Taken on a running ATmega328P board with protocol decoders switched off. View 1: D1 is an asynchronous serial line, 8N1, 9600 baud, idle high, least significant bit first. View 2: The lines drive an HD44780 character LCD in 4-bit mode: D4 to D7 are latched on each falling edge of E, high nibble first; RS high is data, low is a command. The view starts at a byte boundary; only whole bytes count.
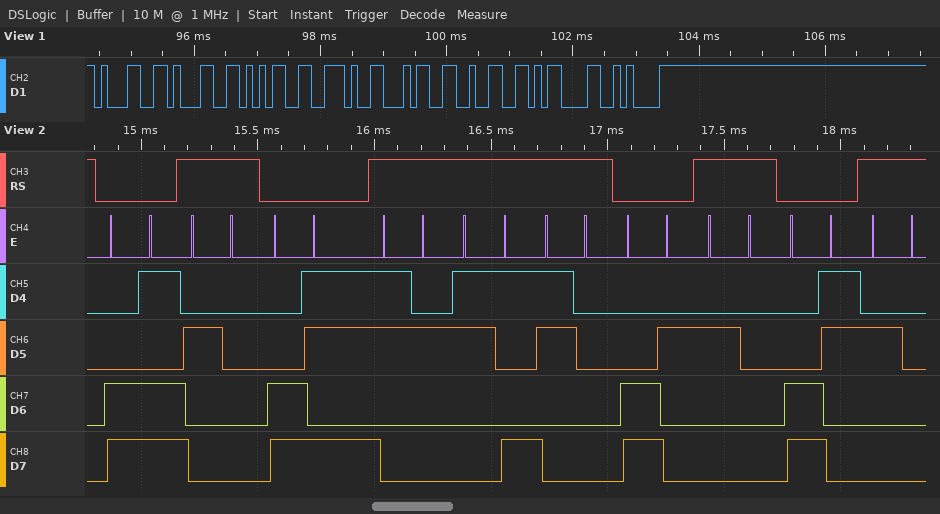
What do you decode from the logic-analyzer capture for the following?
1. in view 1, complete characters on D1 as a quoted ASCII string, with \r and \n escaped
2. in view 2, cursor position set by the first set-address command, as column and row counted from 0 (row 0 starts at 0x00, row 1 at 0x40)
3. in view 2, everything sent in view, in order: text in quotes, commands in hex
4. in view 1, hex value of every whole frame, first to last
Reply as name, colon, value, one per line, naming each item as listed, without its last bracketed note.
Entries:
in view 1, complete characters on D1 as a quoted ASCII string, with \r and \n escaped: "115.42\r\n"
in view 2, cursor position set by the first set-address command, as column and row counted from 0: column 13, row 1
in view 2, everything sent in view, in order: text in quotes, commands in hex: 0xCD " " 0xCB "290" 0xC2 " " 0xC3 " "
in view 1, hex value of every whole frame, first to last: 31 31 35 2E 34 32 0D 0A
